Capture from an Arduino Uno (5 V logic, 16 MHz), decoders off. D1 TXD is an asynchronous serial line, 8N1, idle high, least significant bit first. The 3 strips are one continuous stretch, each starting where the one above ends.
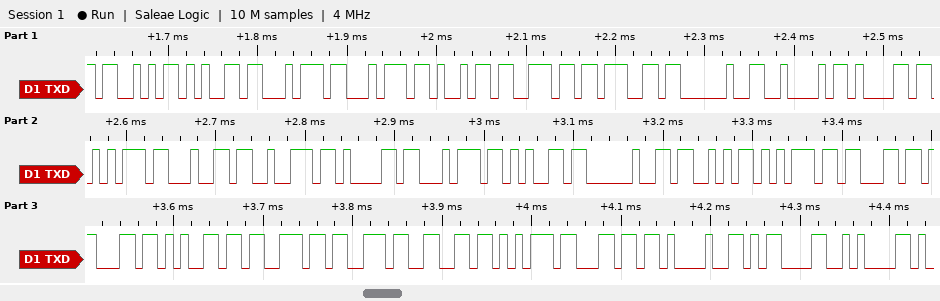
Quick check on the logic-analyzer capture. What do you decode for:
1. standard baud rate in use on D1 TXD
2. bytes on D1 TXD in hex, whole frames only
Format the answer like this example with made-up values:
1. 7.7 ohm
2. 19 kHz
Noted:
1. 115200 baud
2. 53 65 74 74 69 6E 67 20 42 61 75 64 72 61 74 65 20 53 75 63 63 65 73 73 66 75 6C 21 0D 0A
